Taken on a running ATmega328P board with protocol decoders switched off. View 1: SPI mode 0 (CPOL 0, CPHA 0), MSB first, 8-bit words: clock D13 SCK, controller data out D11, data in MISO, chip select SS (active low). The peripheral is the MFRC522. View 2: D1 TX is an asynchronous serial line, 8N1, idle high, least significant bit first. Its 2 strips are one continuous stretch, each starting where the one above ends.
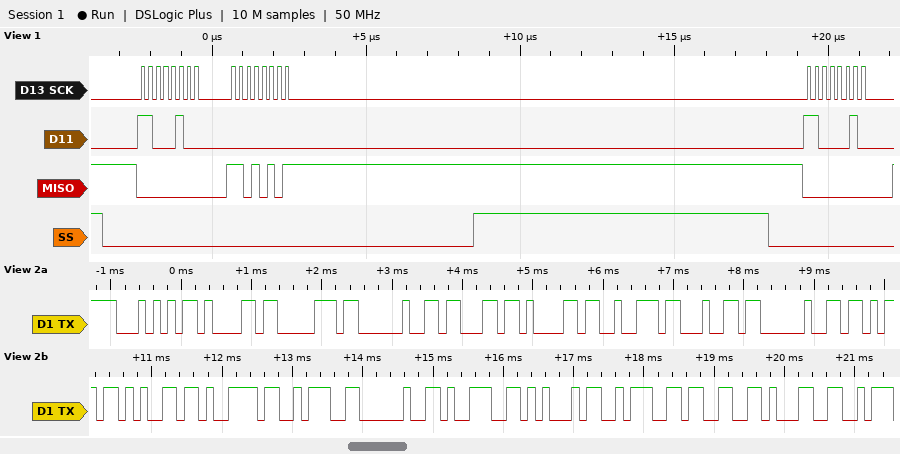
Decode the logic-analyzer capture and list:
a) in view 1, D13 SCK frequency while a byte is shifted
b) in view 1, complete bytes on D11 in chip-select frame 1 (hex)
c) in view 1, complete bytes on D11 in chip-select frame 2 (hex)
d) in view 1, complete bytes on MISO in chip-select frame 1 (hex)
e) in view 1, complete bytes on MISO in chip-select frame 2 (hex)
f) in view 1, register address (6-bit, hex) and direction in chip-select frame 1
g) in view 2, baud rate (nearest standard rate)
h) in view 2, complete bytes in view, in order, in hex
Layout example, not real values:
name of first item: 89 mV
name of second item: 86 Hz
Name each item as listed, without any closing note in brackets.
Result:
in view 1, D13 SCK frequency while a byte is shifted: 4 MHz
in view 1, complete bytes on D11 in chip-select frame 1: C4 00
in view 1, complete bytes on D11 in chip-select frame 2: C2
in view 1, complete bytes on MISO in chip-select frame 1: 00 D5
in view 1, complete bytes on MISO in chip-select frame 2: 00
in view 1, register address (6-bit, hex) and direction in chip-select frame 1: 0x22 read
in view 2, baud rate: 9600 baud
in view 2, complete bytes in view, in order, in hex: 54 61 70 20 63 61 72 64 20 6B 65 79 3A 20 39 45 3A 33 31
